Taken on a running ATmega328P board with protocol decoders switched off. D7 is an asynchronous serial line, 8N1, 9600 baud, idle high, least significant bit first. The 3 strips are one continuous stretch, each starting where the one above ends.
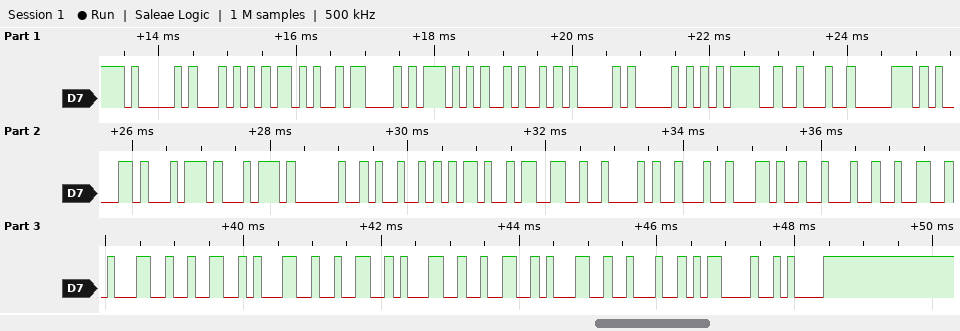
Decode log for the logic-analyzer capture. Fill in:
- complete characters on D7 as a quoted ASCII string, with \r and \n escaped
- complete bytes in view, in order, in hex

"AT+CWJAP=\"patt I-3B\",\"21212121\"\r\n"
41 54 2B 43 57 4A 41 50 3D 22 70 61 74 74 20 49 2D 33 42 22 2C 22 32 31 32 31 32 31 32 31 22 0D 0A
